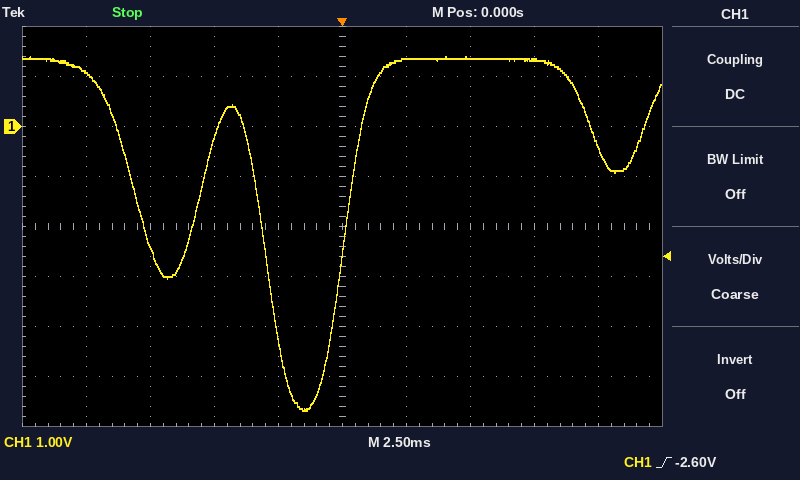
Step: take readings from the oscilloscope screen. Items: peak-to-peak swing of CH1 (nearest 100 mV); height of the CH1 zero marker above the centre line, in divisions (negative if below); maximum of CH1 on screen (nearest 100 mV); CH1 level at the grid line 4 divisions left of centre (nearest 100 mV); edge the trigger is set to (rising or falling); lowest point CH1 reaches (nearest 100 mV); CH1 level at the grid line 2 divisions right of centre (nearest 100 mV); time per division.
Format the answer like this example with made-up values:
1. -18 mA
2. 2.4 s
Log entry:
1. 7.1 V
2. +2.0 div
3. 1.4 V
4. 1.1 V
5. rising
6. -5.7 V
7. 1.4 V
8. 2.5 ms
